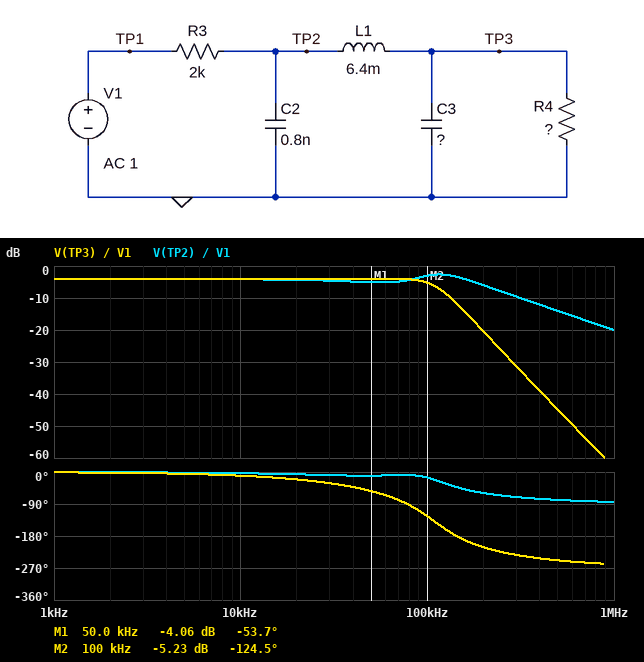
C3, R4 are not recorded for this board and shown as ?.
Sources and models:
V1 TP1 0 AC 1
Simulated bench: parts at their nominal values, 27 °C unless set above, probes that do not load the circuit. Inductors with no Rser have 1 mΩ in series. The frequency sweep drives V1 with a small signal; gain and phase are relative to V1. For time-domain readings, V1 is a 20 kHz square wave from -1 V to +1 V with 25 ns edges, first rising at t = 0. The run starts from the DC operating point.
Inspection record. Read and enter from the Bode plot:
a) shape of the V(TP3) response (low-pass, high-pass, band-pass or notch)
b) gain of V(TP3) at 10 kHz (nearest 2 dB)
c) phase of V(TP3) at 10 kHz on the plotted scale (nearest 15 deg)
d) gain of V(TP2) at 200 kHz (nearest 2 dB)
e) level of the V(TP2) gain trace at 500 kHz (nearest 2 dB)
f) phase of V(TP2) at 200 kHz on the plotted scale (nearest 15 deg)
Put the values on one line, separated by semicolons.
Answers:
low-pass; -4 dB; -15 deg; -6 dB; -14 dB; -60 deg
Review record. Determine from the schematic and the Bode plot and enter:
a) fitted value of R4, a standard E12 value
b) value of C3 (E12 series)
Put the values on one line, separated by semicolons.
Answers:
3.3 kΩ; 560 pF
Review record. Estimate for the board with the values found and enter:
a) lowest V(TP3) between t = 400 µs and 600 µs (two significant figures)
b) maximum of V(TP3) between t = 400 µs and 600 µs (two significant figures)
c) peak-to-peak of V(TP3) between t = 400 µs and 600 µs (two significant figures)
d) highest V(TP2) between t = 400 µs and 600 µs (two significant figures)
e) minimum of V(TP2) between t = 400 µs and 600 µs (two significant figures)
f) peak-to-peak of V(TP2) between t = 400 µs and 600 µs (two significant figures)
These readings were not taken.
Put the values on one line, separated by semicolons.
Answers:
-750 mV; 750 mV; 1.5 V; 700 mV; -700 mV; 1.4 V
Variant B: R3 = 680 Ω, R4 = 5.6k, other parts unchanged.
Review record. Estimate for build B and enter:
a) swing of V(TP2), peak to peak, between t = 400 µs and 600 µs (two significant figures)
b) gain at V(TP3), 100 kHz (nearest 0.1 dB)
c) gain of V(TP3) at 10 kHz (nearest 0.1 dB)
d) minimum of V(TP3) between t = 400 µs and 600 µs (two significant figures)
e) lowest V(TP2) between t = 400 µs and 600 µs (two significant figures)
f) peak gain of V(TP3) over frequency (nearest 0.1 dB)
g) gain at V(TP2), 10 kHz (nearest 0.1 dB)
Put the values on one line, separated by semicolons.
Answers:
1.9 V; 0.2 dB; -0.9 dB; -1.4 V; -940 mV; 2.0 dB; -1.0 dB
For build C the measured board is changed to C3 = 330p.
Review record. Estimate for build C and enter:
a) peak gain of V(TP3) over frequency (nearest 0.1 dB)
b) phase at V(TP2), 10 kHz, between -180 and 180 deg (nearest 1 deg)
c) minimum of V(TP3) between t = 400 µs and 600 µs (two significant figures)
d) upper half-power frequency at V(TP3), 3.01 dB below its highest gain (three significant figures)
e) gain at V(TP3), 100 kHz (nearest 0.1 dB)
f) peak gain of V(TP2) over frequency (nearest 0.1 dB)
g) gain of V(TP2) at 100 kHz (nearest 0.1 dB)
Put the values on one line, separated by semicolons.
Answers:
-4.1 dB; -2 deg; -710 mV; 123 kHz; -5.4 dB; -3.4 dB; -3.6 dB
